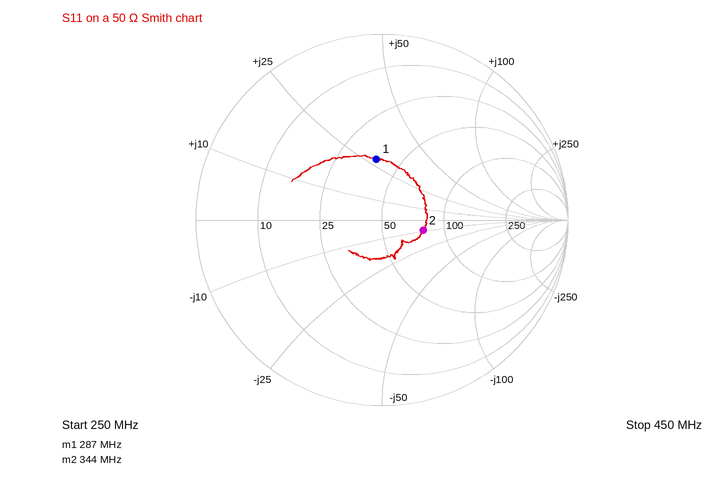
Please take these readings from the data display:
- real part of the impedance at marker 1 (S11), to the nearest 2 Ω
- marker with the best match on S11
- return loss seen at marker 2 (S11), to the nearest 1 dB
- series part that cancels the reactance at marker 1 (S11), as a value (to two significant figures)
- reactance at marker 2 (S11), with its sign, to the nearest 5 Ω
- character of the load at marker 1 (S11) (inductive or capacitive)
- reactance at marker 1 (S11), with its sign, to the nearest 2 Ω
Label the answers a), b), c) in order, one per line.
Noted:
a) 38 Ω
b) marker 2
c) 13 dB
d) 20 pF
e) -10 Ω
f) inductive
g) +28 Ω
